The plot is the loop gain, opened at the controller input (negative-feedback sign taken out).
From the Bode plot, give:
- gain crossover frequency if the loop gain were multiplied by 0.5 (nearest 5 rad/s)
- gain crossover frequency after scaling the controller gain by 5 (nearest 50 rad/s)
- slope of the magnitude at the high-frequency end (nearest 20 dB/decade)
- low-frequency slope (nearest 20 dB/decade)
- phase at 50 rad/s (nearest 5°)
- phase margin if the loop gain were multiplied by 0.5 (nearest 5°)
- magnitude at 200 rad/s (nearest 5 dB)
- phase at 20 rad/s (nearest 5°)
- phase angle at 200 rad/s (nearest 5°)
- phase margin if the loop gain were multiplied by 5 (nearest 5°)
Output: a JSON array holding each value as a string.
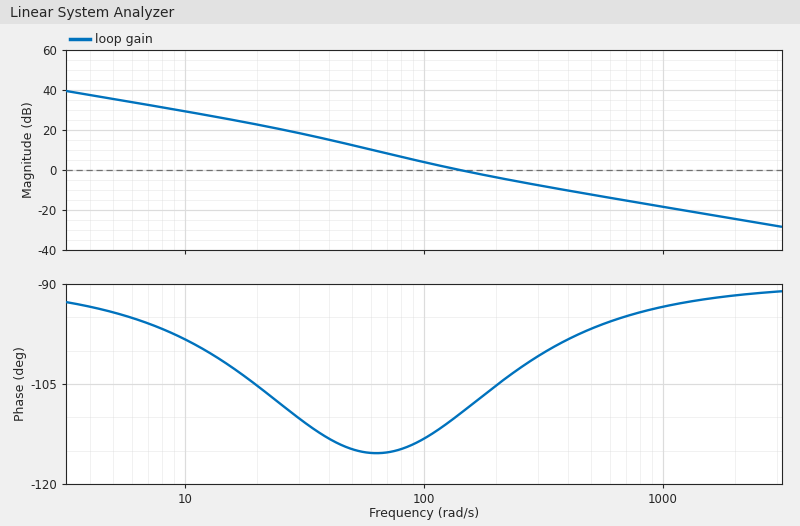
["85 rad/s", "600 rad/s", "-20 dB/decade", "-20 dB/decade", "-115°", "65°", "-5 dB", "-105°", "-105°", "85°"]
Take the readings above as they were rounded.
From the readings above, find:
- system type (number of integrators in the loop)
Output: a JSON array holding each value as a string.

["1"]
